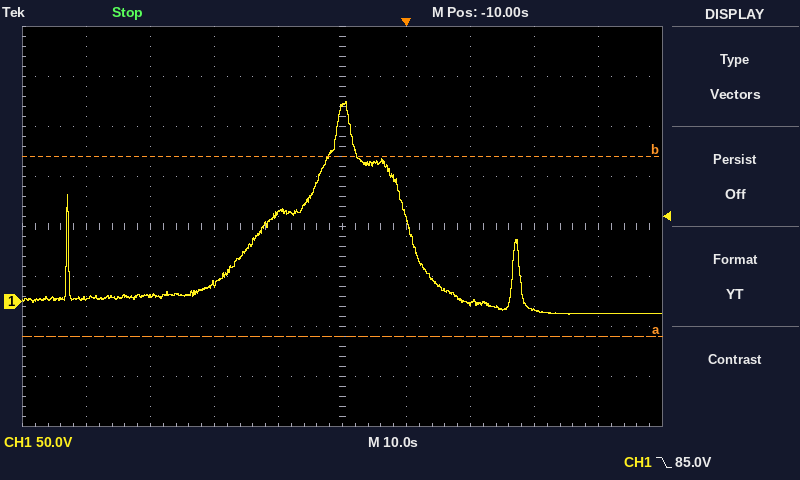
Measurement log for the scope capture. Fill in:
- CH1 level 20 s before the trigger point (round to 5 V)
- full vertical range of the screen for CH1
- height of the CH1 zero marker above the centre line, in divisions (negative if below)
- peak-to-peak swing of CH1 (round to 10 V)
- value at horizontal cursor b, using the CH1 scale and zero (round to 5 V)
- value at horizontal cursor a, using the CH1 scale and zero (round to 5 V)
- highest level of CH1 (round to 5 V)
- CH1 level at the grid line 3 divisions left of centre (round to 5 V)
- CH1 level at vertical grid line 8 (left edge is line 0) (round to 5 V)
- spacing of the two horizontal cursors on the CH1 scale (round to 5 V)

90 V
400 V
-1.5 div
210 V
145 V
-35 V
200 V
5 V
-10 V
180 V
